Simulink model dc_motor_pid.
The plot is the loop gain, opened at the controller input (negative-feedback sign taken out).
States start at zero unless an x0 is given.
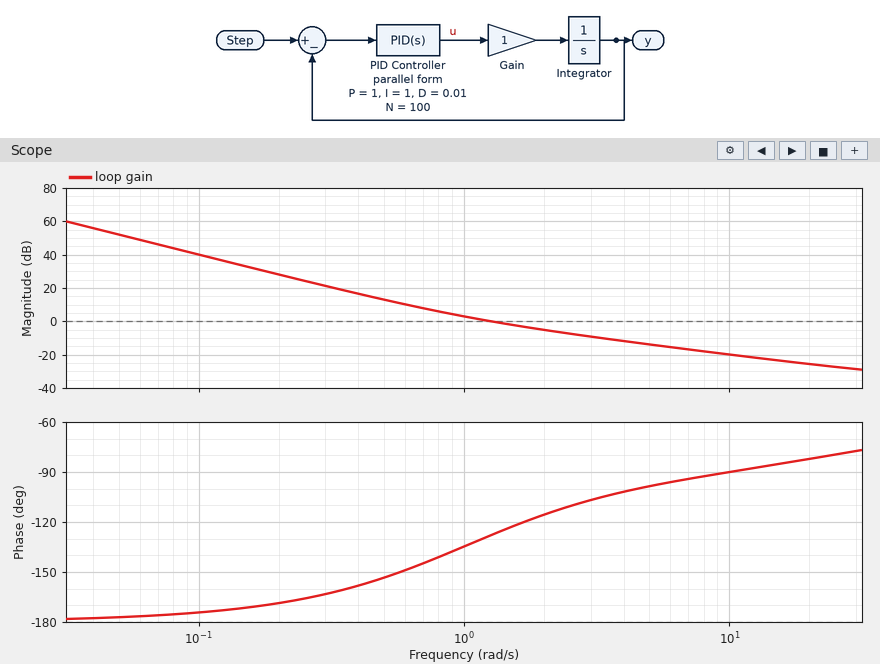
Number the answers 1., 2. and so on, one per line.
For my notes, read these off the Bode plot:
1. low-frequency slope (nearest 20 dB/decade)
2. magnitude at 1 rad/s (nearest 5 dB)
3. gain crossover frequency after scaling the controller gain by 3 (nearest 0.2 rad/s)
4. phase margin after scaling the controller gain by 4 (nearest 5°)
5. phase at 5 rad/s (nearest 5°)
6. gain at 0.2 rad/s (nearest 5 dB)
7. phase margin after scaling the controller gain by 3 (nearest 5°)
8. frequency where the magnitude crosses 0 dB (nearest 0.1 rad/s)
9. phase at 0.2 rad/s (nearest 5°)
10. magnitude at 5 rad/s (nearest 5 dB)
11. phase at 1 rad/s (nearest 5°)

1. -40 dB/decade
2. 5 dB
3. 3.2 rad/s
4. 80°
5. -100°
6. 30 dB
7. 75°
8. 1.3 rad/s
9. -170°
10. -15 dB
11. -135°
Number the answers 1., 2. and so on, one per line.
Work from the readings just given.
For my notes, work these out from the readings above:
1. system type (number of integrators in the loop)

1. 2
